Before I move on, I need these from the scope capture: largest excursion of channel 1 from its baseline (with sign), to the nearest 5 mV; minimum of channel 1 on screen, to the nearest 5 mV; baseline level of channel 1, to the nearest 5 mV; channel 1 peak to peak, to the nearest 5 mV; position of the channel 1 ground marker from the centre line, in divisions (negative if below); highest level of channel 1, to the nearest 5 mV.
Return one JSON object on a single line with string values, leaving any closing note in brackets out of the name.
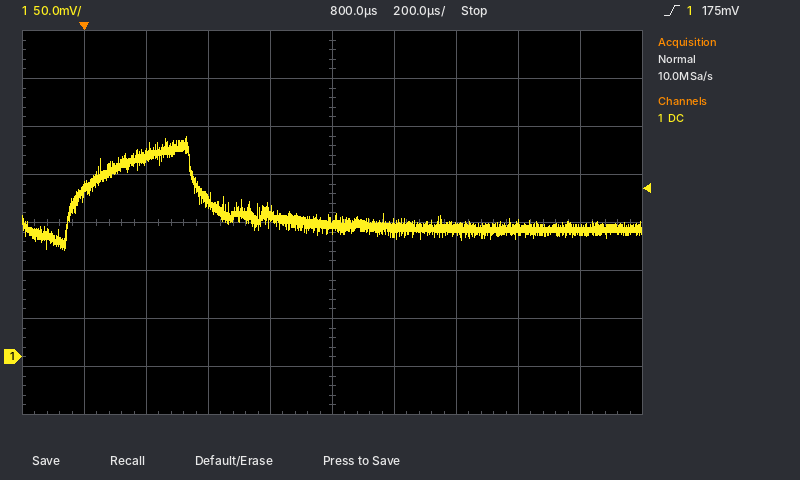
{"largest excursion of channel 1 from its baseline (with sign), to the nearest 5 mV": "+95 mV", "minimum of channel 1 on screen, to the nearest 5 mV": "110 mV", "baseline level of channel 1, to the nearest 5 mV": "135 mV", "channel 1 peak to peak, to the nearest 5 mV": "120 mV", "position of the channel 1 ground marker from the centre line, in divisions": "-2.8 div", "highest level of channel 1, to the nearest 5 mV": "230 mV"}
